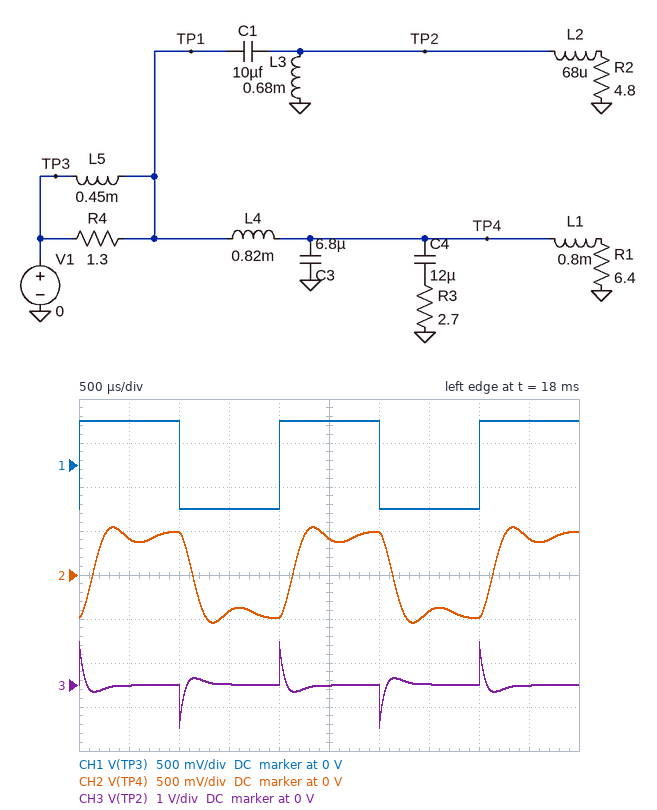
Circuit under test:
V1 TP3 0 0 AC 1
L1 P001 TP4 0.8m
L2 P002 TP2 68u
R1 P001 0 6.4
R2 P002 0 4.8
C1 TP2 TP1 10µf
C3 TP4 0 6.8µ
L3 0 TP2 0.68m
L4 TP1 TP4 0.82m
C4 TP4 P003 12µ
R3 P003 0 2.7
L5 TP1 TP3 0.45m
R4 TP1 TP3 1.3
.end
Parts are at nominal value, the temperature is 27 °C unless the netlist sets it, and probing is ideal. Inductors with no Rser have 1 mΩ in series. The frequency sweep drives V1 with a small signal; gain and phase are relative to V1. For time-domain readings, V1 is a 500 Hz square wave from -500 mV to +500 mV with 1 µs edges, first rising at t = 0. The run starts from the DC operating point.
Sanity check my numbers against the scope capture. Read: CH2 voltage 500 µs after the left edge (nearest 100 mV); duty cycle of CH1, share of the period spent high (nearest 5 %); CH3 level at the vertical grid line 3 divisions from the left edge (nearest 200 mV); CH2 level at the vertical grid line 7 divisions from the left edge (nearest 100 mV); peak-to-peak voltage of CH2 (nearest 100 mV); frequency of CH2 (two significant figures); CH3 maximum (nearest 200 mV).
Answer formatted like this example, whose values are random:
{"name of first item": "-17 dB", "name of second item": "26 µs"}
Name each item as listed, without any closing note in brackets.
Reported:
{"CH2 voltage 500 µs after the left edge": "400 mV", "duty cycle of CH1, share of the period spent high": "50 %", "CH3 level at the vertical grid line 3 divisions from the left edge": "0 V", "CH2 level at the vertical grid line 7 divisions from the left edge": "-400 mV", "peak-to-peak voltage of CH2": "1.1 V", "frequency of CH2": "500 Hz", "CH3 maximum": "1.0 V"}
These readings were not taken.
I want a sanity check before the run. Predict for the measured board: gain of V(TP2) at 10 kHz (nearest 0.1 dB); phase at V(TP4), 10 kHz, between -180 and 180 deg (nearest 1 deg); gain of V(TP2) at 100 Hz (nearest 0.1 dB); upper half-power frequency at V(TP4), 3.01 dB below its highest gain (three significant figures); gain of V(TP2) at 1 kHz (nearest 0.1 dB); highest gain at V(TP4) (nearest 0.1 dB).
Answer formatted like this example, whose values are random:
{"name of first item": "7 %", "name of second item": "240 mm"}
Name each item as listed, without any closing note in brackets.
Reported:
{"gain of V(TP2) at 10 kHz": "-0.2 dB", "phase at V(TP4), 10 kHz, between -180 and 180 deg": "-143 deg", "gain of V(TP2) at 100 Hz": "-51.5 dB", "upper half-power frequency at V(TP4), 3.01 dB below its highest gain": "2.03 kHz", "gain of V(TP2) at 1 kHz": "-14.0 dB", "highest gain at V(TP4)": "0.2 dB"}
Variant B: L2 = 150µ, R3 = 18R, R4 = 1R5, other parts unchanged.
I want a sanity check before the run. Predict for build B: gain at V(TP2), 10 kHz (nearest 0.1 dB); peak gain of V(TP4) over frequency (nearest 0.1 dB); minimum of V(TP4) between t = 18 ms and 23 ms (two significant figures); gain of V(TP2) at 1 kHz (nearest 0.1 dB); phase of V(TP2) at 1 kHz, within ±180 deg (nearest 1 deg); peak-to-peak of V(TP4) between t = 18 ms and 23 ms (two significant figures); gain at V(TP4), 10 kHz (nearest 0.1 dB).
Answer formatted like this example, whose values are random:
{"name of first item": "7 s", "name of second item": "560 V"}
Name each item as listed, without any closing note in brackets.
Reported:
{"gain at V(TP2), 10 kHz": "0.6 dB", "peak gain of V(TP4) over frequency": "0 dB", "minimum of V(TP4) between t = 18 ms and 23 ms": "-480 mV", "gain of V(TP2) at 1 kHz": "-14.2 dB", "phase of V(TP2) at 1 kHz, within ±180 deg": "133 deg", "peak-to-peak of V(TP4) between t = 18 ms and 23 ms": "950 mV", "gain at V(TP4), 10 kHz": "-27.2 dB"}
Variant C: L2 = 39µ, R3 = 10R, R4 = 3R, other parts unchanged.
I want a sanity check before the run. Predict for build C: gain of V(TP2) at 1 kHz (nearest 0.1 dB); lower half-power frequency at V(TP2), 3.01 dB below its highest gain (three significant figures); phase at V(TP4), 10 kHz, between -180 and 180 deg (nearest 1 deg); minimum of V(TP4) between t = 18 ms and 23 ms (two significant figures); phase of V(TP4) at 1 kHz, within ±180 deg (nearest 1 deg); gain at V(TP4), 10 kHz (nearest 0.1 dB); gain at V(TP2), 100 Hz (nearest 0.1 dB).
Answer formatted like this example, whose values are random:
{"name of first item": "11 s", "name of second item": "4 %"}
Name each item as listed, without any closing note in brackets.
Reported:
{"gain of V(TP2) at 1 kHz": "-14.1 dB", "lower half-power frequency at V(TP2), 3.01 dB below its highest gain": "13.0 kHz", "phase at V(TP4), 10 kHz, between -180 and 180 deg": "-160 deg", "minimum of V(TP4) between t = 18 ms and 23 ms": "-480 mV", "phase of V(TP4) at 1 kHz, within ±180 deg": "-46 deg", "gain at V(TP4), 10 kHz": "-31.1 dB", "gain at V(TP2), 100 Hz": "-51.5 dB"}
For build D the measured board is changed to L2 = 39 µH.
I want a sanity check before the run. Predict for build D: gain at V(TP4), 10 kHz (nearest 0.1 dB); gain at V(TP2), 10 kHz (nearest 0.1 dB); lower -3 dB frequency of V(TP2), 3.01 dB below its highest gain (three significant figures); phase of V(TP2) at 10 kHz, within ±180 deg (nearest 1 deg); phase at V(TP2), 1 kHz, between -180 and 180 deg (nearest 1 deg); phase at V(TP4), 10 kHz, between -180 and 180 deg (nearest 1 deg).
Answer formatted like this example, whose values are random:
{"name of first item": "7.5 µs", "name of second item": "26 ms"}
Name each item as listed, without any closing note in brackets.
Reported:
{"gain at V(TP4), 10 kHz": "-32.2 dB", "gain at V(TP2), 10 kHz": "-1.0 dB", "lower -3 dB frequency of V(TP2), 3.01 dB below its highest gain": "2.91 kHz", "phase of V(TP2) at 10 kHz, within ±180 deg": "22 deg", "phase at V(TP2), 1 kHz, between -180 and 180 deg": "126 deg", "phase at V(TP4), 10 kHz, between -180 and 180 deg": "-147 deg"}
